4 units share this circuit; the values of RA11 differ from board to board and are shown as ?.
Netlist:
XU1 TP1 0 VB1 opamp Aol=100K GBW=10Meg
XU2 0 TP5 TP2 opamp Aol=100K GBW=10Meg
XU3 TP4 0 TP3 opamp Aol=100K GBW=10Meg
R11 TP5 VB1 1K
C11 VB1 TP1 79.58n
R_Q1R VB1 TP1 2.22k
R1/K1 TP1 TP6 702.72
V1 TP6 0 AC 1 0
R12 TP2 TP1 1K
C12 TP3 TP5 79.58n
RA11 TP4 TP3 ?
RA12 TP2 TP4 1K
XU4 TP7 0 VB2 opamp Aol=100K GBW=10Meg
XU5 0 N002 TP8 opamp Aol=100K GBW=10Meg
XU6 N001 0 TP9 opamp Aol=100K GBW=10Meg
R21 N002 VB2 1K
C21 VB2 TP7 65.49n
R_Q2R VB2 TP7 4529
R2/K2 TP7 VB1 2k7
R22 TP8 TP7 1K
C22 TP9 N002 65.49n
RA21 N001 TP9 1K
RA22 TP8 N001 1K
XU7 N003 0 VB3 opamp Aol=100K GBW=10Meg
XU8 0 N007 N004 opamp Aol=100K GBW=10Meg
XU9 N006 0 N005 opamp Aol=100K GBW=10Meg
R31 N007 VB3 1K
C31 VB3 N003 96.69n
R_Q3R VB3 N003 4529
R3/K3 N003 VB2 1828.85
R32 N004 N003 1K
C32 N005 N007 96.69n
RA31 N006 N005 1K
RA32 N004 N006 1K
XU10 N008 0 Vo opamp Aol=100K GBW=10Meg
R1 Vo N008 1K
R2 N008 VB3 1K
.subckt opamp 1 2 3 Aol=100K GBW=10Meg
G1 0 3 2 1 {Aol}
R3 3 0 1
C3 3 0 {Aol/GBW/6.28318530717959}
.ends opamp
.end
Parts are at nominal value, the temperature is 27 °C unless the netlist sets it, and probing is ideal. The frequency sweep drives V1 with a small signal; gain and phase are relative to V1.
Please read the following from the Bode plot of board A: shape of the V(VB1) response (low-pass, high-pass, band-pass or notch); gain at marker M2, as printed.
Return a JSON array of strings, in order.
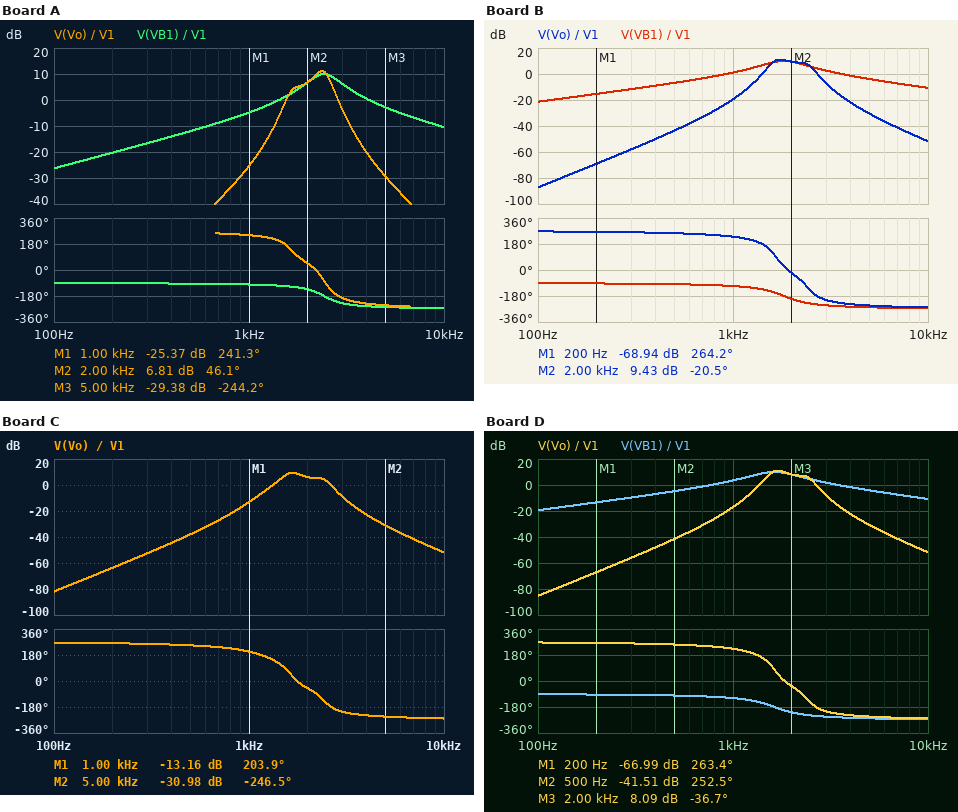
["band-pass", "6.81 dB"]
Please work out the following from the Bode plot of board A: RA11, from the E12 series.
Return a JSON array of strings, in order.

["680 Ω"]
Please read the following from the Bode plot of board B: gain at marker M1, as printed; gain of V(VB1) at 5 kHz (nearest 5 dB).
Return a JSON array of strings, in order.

["-68.94 dB", "-5 dB"]
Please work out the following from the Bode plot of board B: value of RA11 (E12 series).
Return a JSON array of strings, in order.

["1.2 kΩ"]
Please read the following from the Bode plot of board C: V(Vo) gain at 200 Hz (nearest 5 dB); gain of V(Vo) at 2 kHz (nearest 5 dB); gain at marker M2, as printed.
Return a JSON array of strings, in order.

["-65 dB", "5 dB", "-30.98 dB"]
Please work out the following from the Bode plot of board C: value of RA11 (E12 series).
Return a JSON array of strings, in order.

["2.2 kΩ"]
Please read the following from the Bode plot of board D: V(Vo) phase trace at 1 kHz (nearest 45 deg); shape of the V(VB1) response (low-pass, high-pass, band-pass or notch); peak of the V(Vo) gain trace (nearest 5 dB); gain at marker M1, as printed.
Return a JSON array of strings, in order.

["225 deg", "band-pass", "10 dB", "-66.99 dB"]
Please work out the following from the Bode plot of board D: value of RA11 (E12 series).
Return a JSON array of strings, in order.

["1.5 kΩ"]
